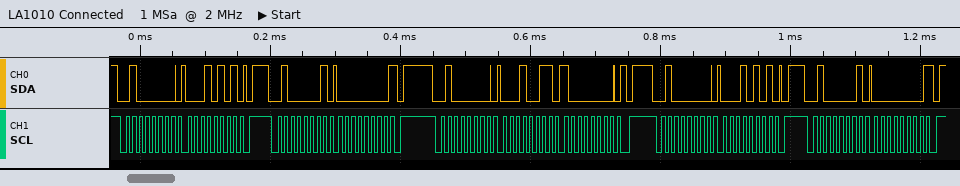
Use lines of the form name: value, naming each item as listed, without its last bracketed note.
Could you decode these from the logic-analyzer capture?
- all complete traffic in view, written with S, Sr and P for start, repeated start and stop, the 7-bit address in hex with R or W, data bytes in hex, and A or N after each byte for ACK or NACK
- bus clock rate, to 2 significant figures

all complete traffic in view, written with S, Sr and P for start, repeated start and stop, the 7-bit address in hex with R or W, data bytes in hex, and A or N after each byte for ACK or NACK: S 20W A 15 A P S 20R A 00 N P S 20W A 13 A 80 A P S 20W A 15 A P S 20R A 00 N P
bus clock rate, to 2 significant figures: 100 kHz
